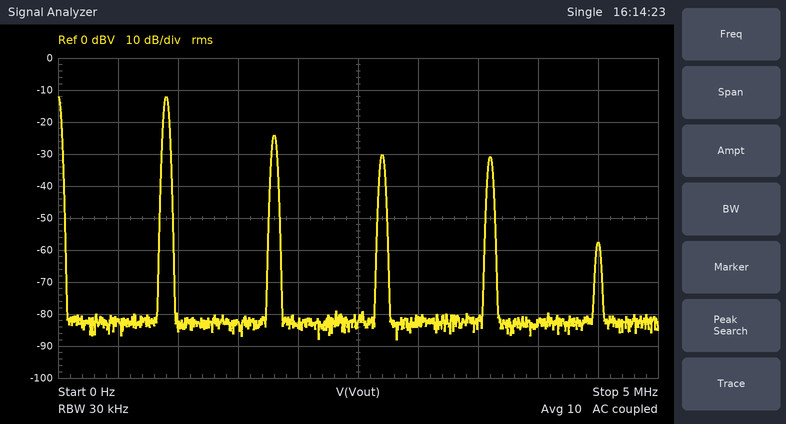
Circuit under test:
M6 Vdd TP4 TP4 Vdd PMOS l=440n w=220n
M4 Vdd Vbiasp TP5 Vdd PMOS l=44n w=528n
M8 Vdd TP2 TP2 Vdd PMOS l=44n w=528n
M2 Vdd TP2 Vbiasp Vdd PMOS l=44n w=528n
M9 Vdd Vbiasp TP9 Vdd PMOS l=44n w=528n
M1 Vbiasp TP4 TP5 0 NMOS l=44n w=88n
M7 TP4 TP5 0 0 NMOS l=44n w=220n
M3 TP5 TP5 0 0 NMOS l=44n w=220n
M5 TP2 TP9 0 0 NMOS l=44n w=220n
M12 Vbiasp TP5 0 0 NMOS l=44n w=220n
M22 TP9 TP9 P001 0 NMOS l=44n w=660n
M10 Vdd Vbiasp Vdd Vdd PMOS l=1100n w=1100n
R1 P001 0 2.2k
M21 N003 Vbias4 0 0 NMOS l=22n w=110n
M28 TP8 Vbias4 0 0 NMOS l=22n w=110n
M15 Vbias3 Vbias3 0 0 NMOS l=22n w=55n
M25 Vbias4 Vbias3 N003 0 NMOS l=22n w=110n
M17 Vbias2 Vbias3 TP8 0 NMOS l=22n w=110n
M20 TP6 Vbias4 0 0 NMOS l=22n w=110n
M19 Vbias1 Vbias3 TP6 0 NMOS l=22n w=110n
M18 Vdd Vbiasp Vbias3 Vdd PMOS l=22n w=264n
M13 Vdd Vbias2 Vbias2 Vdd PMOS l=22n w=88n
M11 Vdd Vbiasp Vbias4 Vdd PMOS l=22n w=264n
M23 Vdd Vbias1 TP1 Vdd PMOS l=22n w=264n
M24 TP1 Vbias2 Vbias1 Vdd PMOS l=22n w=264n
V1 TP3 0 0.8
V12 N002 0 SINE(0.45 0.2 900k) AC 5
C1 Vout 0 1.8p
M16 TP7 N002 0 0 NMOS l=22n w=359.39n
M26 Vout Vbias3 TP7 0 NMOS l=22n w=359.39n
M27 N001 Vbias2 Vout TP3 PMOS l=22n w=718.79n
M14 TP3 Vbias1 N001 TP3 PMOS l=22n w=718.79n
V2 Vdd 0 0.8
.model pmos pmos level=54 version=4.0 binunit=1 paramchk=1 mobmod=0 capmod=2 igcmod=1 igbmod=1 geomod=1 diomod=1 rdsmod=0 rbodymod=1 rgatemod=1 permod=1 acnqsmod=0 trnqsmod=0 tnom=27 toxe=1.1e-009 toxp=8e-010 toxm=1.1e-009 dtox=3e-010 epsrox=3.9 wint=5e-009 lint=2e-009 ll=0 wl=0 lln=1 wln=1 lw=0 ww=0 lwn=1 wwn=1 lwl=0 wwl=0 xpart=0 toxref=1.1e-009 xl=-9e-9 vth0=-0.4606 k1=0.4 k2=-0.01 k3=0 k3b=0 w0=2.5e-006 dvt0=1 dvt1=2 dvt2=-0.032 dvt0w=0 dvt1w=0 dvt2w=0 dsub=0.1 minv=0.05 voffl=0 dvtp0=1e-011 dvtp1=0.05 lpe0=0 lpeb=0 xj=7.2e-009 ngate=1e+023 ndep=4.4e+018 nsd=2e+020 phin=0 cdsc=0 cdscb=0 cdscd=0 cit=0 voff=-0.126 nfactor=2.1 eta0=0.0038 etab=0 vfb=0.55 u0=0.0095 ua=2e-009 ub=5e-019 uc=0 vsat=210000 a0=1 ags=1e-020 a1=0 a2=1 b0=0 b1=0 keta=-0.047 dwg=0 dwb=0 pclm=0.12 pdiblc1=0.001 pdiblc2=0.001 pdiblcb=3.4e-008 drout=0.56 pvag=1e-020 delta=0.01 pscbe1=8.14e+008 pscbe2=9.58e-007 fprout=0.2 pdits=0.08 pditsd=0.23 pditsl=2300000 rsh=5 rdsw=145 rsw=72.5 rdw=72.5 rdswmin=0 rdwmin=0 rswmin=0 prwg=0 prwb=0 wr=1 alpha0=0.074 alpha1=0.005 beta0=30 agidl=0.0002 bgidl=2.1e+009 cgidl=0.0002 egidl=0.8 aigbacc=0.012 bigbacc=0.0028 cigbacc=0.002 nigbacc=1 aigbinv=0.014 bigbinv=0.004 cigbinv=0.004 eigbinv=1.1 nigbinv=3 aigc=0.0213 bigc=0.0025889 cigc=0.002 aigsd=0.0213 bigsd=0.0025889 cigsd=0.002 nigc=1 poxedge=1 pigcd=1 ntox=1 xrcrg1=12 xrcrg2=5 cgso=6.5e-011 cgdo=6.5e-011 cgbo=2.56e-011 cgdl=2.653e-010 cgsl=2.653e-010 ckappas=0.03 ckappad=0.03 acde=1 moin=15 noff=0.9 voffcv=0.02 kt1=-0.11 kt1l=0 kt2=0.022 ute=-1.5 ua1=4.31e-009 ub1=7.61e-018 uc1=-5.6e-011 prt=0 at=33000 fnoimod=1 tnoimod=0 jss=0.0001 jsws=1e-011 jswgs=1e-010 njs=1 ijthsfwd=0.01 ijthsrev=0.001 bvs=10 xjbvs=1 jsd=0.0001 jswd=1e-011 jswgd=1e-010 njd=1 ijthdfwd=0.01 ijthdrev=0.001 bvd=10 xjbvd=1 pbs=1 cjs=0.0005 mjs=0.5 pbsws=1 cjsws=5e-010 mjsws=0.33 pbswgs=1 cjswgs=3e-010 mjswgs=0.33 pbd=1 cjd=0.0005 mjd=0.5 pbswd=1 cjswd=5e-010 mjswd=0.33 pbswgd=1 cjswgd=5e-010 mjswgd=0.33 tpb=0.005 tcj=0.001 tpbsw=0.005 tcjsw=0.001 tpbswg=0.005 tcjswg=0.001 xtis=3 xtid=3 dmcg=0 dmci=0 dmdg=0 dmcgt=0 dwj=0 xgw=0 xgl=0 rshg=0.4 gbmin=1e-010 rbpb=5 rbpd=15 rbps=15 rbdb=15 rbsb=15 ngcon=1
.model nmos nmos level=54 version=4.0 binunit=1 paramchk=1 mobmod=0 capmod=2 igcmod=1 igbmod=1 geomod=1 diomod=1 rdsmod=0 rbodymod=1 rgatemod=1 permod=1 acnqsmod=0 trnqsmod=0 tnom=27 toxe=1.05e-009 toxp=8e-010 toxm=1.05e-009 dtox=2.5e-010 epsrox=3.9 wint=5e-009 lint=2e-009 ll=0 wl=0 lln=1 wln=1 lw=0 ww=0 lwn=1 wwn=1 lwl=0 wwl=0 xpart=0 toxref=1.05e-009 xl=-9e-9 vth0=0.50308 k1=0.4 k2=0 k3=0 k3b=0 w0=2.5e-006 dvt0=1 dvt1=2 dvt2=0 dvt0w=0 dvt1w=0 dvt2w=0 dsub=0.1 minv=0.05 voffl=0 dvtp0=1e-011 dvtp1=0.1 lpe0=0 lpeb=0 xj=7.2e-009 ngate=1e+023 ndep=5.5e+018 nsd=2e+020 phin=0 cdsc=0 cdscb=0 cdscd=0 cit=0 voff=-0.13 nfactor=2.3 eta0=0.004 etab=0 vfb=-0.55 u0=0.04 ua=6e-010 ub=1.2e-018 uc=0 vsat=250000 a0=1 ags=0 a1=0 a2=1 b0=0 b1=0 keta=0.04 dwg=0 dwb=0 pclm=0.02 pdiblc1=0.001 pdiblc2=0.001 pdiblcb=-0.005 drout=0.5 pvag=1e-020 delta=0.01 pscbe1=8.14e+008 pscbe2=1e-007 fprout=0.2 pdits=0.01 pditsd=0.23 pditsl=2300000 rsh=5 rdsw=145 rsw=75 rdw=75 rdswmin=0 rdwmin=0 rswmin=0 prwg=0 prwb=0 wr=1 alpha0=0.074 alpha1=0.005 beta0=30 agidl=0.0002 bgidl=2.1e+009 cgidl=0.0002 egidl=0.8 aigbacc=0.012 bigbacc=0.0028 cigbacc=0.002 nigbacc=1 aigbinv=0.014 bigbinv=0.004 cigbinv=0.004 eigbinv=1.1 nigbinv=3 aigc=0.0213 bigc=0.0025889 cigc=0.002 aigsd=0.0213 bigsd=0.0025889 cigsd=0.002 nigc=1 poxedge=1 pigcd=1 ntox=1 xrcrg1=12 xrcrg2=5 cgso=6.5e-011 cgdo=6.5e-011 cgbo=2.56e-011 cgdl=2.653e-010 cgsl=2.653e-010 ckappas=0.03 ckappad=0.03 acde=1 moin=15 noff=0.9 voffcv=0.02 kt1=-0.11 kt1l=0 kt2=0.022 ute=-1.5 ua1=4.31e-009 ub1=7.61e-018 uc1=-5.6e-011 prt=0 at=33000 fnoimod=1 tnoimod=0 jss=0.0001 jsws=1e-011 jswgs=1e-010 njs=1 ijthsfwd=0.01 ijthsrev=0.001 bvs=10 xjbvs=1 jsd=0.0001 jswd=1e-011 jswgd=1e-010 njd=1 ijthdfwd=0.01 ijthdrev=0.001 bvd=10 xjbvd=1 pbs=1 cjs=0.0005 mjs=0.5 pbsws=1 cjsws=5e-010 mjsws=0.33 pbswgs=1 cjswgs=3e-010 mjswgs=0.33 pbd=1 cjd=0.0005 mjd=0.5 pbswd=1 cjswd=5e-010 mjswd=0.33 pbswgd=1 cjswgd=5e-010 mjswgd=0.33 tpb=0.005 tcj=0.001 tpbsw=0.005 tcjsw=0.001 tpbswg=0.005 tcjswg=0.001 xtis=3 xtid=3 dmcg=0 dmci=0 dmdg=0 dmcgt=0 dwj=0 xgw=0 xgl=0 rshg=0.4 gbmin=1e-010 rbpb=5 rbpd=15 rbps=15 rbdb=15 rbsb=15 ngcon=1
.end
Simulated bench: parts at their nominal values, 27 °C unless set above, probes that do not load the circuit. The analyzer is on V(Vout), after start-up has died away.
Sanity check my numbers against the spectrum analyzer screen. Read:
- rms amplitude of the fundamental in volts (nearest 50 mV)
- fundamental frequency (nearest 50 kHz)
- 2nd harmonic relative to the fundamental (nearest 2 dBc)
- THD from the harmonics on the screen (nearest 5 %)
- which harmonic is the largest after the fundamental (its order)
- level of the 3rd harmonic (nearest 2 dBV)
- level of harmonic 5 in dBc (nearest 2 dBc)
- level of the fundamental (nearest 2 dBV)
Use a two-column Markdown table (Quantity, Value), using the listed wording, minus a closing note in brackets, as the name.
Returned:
| Quantity | Value |
|---|---|
| rms amplitude of the fundamental in volts | 250 mV |
| fundamental frequency | 900 kHz |
| 2nd harmonic relative to the fundamental | -12 dBc |
| THD from the harmonics on the screen | 30 % |
| which harmonic is the largest after the fundamental | 2 |
| level of the 3rd harmonic | -30 dBV |
| level of harmonic 5 in dBc | -46 dBc |
| level of the fundamental | -12 dBV |
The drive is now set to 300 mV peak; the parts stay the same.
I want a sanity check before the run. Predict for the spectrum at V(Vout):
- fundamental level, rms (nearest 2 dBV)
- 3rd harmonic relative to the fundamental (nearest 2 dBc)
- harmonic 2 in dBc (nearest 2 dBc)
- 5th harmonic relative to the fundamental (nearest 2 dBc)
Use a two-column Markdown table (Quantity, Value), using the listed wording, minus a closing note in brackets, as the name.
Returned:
| Quantity | Value |
|---|---|
| fundamental level, rms | -12 dBV |
| 3rd harmonic relative to the fundamental | -14 dBc |
| harmonic 2 in dBc | -14 dBc |
| 5th harmonic relative to the fundamental | -26 dBc |
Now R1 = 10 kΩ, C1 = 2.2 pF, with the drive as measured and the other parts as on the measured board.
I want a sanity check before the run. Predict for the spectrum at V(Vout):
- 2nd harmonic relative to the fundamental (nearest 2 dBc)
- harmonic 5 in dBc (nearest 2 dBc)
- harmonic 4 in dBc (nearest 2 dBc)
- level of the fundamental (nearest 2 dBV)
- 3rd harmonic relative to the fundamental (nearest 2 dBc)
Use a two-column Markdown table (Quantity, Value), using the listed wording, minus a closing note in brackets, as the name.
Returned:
| Quantity | Value |
|---|---|
| 2nd harmonic relative to the fundamental | -18 dBc |
| harmonic 5 in dBc | -26 dBc |
| harmonic 4 in dBc | -26 dBc |
| level of the fundamental | -12 dBV |
| 3rd harmonic relative to the fundamental | -14 dBc |
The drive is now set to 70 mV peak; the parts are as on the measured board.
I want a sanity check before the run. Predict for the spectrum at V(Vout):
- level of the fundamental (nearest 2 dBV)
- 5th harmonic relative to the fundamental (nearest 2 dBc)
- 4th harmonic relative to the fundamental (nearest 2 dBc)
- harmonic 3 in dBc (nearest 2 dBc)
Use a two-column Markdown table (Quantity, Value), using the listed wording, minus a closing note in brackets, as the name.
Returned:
| Quantity | Value |
|---|---|
| level of the fundamental | -20 dBV |
| 5th harmonic relative to the fundamental | -40 dBc |
| 4th harmonic relative to the fundamental | -38 dBc |
| harmonic 3 in dBc | -28 dBc |
